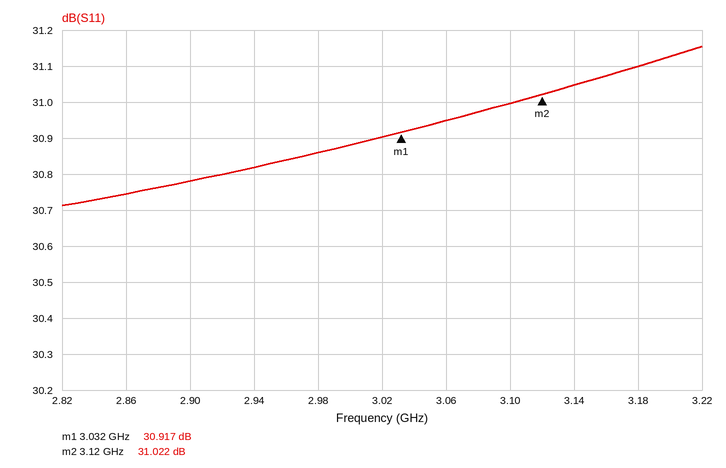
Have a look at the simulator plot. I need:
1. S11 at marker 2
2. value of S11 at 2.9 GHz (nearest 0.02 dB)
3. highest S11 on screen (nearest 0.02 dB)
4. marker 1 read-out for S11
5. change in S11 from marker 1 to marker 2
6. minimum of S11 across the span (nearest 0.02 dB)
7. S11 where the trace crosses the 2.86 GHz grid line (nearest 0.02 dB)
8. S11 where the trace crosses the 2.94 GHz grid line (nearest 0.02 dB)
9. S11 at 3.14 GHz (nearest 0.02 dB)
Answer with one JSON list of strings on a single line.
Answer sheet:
["31.022 dB", "30.78 dB", "31.16 dB", "30.917 dB", "0.105 dB", "30.72 dB", "30.74 dB", "30.82 dB", "31.04 dB"]
